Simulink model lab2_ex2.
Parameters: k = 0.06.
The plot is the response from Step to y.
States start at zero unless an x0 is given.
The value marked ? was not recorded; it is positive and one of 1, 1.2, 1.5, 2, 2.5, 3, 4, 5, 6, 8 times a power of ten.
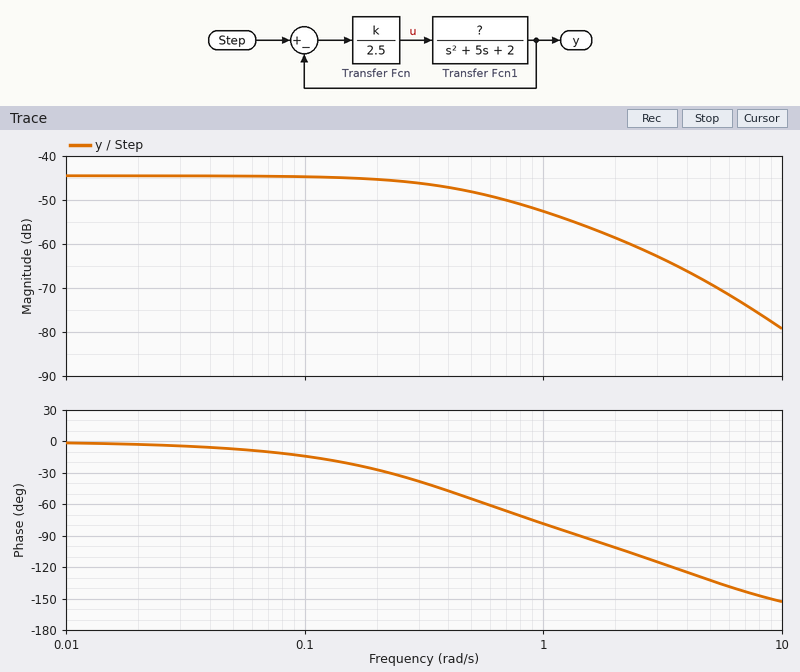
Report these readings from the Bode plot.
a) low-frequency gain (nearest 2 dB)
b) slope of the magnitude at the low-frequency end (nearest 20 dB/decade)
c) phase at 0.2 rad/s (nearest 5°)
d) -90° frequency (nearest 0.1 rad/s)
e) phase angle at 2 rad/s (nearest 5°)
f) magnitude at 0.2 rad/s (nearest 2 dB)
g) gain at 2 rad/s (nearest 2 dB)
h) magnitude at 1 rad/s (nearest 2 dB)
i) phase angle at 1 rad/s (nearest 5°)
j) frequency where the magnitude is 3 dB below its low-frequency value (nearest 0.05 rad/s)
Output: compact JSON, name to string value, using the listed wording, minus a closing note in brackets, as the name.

{"low-frequency gain": "-44 dB", "slope of the magnitude at the low-frequency end": "0 dB/decade", "phase at 0.2 rad/s": "-25°", "-90° frequency": "1.4 rad/s", "phase angle at 2 rad/s": "-100°", "magnitude at 0.2 rad/s": "-46 dB", "gain at 2 rad/s": "-58 dB", "magnitude at 1 rad/s": "-52 dB", "phase angle at 1 rad/s": "-80°", "frequency where the magnitude is 3 dB below its low-frequency value": "0.45 rad/s"}
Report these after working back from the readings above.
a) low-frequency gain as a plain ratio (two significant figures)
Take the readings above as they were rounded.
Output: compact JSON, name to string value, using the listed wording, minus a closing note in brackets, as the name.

{"low-frequency gain as a plain ratio": "0.0063"}
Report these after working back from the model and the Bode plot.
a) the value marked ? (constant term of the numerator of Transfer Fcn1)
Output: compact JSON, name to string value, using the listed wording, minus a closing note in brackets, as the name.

{"the value marked ?": "0.5"}
